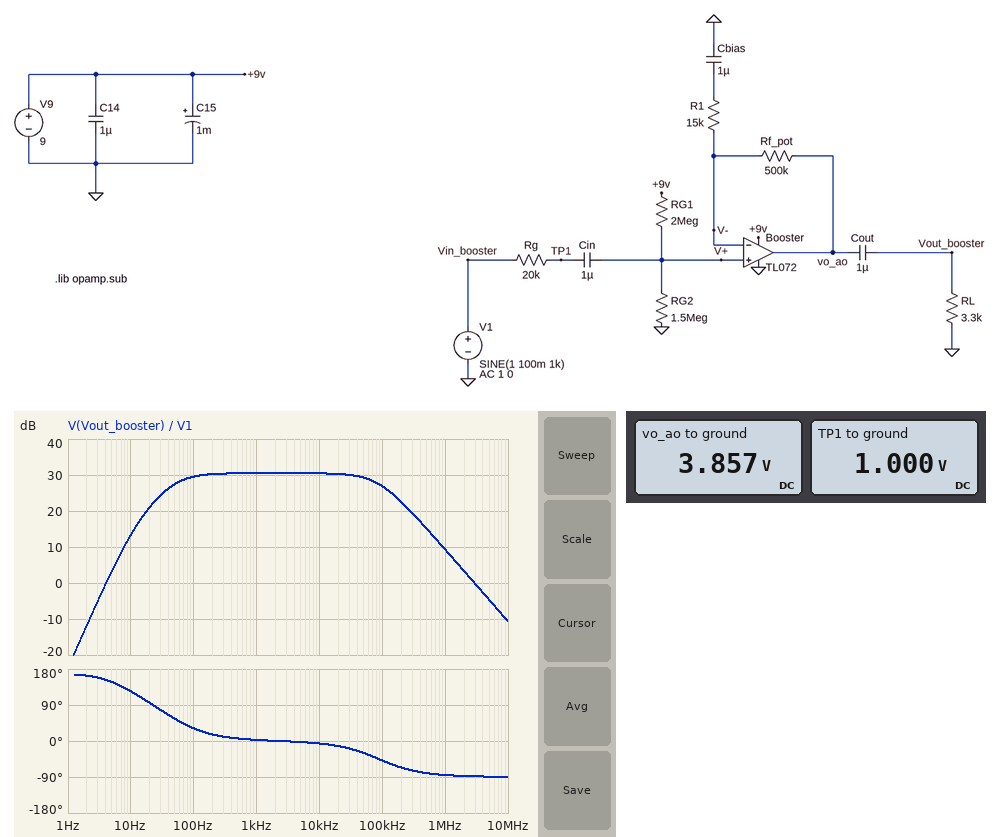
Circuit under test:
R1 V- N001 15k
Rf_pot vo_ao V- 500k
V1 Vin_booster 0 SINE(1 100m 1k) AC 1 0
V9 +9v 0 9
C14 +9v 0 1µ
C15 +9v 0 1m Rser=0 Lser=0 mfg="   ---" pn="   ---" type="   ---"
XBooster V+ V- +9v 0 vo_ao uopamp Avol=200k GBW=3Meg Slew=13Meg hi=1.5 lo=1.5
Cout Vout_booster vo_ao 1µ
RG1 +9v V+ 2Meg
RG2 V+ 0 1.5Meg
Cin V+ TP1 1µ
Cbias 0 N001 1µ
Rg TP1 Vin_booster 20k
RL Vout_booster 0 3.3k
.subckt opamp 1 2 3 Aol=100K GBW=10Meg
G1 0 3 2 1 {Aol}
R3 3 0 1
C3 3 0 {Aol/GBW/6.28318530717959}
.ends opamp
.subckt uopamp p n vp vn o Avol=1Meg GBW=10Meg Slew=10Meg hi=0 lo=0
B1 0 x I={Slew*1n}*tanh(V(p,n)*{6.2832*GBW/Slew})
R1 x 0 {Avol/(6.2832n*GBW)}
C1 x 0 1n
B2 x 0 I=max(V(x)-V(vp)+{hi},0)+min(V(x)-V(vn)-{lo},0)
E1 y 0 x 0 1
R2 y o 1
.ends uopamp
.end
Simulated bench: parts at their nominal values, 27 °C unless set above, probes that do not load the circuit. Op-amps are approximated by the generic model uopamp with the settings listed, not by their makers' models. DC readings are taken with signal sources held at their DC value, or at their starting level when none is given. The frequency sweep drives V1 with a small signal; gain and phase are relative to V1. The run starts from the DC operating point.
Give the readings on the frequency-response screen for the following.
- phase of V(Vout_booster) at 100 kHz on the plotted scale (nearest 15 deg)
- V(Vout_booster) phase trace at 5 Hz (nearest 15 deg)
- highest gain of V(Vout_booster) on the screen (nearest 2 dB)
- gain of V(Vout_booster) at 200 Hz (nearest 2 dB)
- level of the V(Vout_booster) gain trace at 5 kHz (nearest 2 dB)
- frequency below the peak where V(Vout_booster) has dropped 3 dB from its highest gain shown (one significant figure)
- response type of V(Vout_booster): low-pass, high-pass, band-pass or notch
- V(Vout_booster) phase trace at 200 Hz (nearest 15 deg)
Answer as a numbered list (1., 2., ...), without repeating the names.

1. -45 deg
2. 150 deg
3. 30 dB
4. 30 dB
5. 30 dB
6. 50 Hz
7. band-pass
8. 15 deg
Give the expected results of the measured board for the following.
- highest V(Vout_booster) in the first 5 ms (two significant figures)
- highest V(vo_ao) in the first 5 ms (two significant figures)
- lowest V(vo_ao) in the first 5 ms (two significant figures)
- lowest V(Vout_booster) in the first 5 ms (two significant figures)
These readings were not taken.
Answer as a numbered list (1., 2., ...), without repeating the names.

1. 3.2 V
2. 7.2 V
3. 1.5 V
4. -2.6 V
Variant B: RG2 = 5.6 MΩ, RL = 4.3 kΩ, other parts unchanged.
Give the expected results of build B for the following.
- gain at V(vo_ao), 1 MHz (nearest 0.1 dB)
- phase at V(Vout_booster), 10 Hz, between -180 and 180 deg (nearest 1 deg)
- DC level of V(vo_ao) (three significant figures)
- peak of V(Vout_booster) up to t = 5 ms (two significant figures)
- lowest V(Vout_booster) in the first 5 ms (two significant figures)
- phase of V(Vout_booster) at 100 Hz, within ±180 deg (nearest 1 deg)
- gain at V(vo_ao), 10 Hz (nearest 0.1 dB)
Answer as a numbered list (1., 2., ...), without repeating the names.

1. 9.4 dB
2. 120 deg
3. 6.63 V
4. 1.3 V
5. -3.3 V
6. 26 deg
7. 27.3 dB
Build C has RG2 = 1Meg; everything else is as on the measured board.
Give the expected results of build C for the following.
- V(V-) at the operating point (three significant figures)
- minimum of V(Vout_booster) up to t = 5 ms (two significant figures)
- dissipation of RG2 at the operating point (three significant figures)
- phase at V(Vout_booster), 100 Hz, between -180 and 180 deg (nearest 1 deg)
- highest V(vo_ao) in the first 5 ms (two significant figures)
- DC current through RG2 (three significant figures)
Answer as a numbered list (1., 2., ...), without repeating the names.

1. 3.00 V
2. -1.9 V
3. 9.00 µW
4. 32 deg
5. 6.3 V
6. 3.00 µA
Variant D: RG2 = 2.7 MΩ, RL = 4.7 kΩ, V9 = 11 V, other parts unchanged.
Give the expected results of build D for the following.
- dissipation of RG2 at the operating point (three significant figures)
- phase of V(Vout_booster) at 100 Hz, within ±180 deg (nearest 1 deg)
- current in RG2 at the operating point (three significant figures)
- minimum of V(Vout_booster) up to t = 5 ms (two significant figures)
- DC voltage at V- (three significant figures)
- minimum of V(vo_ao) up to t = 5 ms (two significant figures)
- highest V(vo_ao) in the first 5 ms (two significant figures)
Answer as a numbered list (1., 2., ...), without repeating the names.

1. 14.8 µW
2. 25 deg
3. 2.34 µA
4. -3.5 V
5. 6.32 V
6. 2.9 V
7. 9.5 V
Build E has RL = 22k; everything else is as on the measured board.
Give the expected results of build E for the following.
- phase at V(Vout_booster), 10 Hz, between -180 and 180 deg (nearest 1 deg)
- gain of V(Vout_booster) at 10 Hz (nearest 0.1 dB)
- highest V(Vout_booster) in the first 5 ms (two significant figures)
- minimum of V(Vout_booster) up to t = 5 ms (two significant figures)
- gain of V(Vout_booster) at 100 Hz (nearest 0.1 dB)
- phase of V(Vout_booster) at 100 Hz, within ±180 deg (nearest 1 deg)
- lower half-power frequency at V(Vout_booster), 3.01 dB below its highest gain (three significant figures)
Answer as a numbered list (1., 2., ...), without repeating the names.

1. 82 deg
2. 25.4 dB
3. 3.3 V
4. -2.4 V
5. 30.4 dB
6. 10 deg
7. 14.0 Hz
